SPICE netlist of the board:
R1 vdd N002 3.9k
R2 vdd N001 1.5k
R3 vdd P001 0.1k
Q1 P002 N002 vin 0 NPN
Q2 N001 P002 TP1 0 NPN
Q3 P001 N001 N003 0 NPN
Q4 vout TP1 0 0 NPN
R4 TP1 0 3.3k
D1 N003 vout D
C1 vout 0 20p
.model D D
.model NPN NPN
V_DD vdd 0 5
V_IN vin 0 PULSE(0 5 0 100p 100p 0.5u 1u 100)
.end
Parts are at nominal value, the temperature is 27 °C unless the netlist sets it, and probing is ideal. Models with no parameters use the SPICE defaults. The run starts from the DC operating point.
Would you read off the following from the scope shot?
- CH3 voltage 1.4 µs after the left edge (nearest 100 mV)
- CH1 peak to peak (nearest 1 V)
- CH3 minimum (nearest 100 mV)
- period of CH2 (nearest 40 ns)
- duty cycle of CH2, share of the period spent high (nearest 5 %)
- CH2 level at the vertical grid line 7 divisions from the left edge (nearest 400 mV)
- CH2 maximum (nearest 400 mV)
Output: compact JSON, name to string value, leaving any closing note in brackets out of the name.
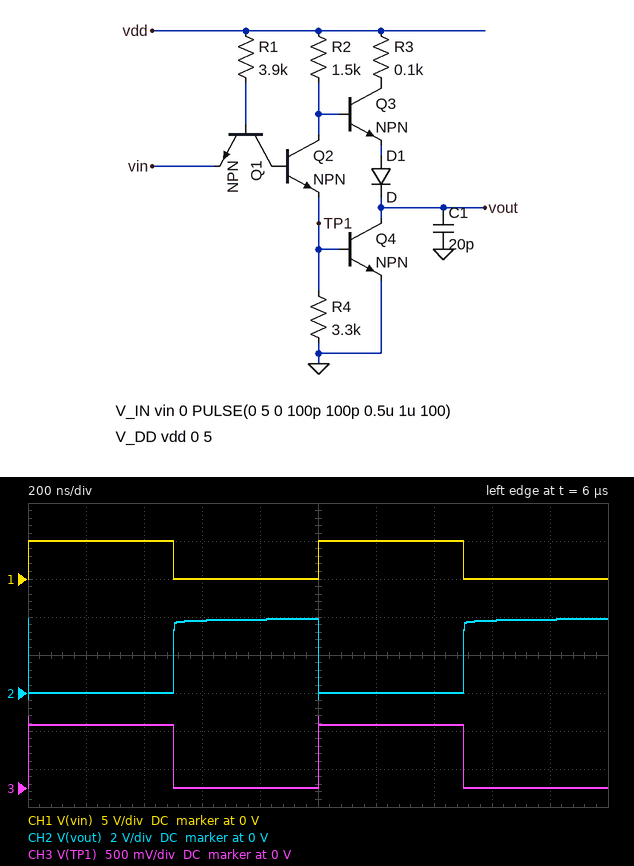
{"CH3 voltage 1.4 µs after the left edge": "800 mV", "CH1 peak to peak": "5 V", "CH3 minimum": "0 V", "period of CH2": "1.00 µs", "duty cycle of CH2, share of the period spent high": "50 %", "CH2 level at the vertical grid line 7 divisions from the left edge": "0 V", "CH2 maximum": "4.0 V"}
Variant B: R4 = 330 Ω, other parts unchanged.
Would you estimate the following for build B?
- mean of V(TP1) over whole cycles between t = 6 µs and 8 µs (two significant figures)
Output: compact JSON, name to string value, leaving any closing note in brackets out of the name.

{"mean of V(TP1) over whole cycles between t = 6 µs and 8 µs": "400 mV"}
